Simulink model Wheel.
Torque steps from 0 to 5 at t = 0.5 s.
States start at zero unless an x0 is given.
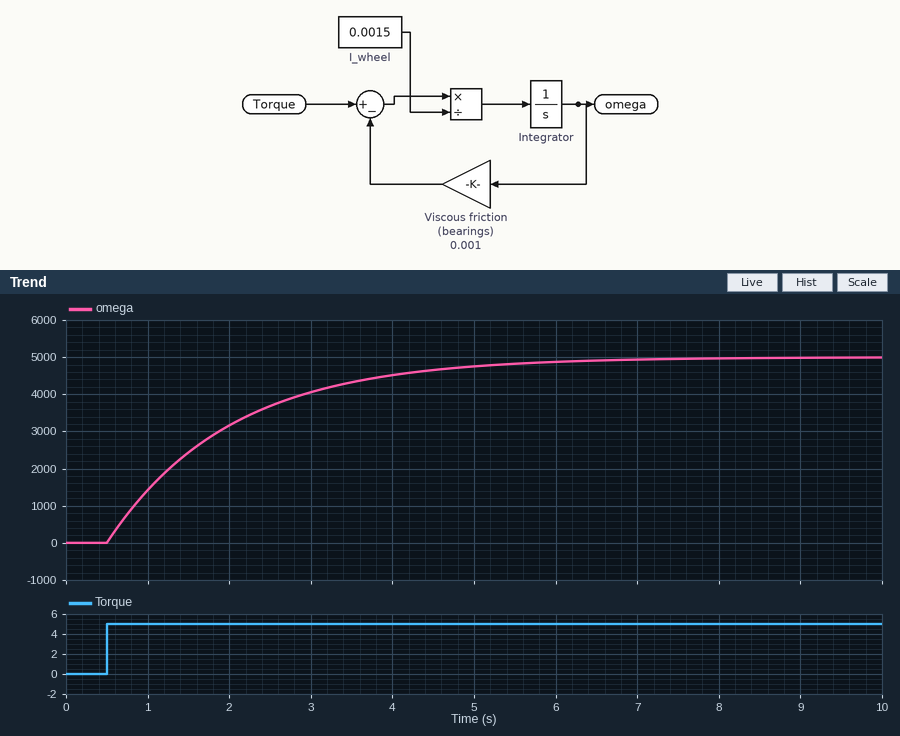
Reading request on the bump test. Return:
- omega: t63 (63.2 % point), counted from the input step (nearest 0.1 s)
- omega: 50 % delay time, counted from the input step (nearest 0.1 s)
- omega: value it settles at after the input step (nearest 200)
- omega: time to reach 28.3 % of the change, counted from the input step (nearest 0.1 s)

1.5 s
1.0 s
5000
0.5 s
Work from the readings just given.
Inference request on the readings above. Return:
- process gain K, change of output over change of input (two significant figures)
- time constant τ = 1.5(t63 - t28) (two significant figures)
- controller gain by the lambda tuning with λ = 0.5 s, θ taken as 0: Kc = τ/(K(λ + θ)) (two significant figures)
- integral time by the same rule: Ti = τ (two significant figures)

1000
1.5 s
0.0030
1.5 s
